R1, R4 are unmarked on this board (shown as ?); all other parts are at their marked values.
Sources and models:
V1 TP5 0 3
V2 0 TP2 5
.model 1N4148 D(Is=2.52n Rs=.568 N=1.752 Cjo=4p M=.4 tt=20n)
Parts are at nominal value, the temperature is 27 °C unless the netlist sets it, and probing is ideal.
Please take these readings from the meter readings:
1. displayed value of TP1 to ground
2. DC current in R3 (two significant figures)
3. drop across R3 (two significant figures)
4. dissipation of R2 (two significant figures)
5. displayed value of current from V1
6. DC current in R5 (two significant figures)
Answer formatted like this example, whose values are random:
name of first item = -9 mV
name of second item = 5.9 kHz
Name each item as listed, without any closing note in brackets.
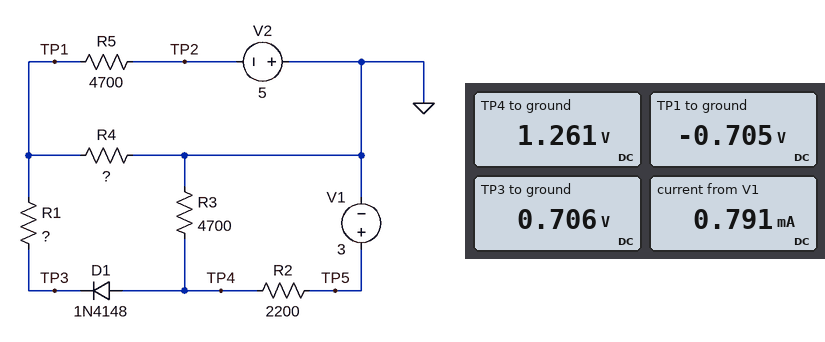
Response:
displayed value of TP1 to ground = -0.705 V
DC current in R3 = 270 µA
drop across R3 = 1.3 V
dissipation of R2 = 1.4 mW
displayed value of current from V1 = 0.791 mA
DC current in R5 = 910 µA
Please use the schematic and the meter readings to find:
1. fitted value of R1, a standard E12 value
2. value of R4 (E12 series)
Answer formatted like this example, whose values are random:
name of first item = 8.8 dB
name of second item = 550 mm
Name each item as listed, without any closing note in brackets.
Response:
fitted value of R1, a standard E12 value = 2.7 kΩ
value of R4 = 1.8 kΩ
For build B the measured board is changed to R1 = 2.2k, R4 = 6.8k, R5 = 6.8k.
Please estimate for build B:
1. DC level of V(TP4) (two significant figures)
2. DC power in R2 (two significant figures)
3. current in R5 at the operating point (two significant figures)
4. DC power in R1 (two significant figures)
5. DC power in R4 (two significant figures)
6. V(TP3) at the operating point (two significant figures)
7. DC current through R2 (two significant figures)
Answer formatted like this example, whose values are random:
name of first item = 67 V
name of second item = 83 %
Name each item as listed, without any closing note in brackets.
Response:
DC level of V(TP4) = 1.2 V
DC power in R2 = 1.5 mW
current in R5 at the operating point = 650 µA
DC power in R1 = 690 µW
DC power in R4 = 51 µW
V(TP3) at the operating point = 640 mV
DC current through R2 = 820 µA
